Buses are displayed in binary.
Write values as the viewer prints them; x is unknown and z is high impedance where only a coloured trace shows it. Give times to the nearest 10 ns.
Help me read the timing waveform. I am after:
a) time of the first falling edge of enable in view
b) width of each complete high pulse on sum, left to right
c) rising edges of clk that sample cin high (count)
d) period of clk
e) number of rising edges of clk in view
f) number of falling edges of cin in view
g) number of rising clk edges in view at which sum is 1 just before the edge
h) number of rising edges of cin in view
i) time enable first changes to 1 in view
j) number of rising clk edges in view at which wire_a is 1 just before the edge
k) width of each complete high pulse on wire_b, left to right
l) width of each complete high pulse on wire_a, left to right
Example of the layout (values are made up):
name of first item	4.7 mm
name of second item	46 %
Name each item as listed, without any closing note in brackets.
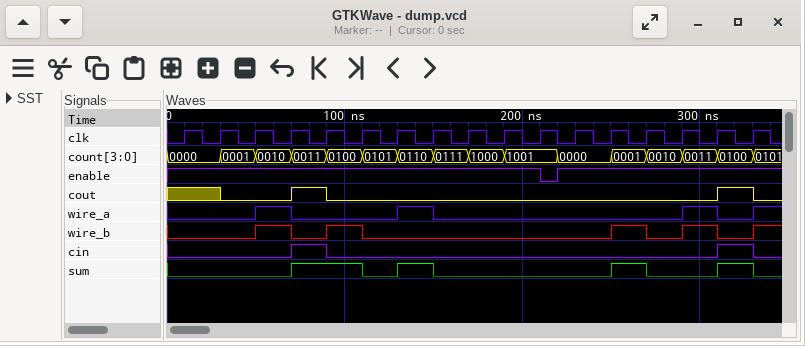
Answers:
time of the first falling edge of enable in view	210 ns
width of each complete high pulse on sum, left to right	40 ns, 20 ns, 20 ns, 20 ns
rising edges of clk that sample cin high	2
period of clk	20 ns
number of rising edges of clk in view	17
number of falling edges of cin in view	2
number of rising clk edges in view at which sum is 1 just before the edge	5
number of rising edges of cin in view	2
time enable first changes to 1 in view	220 ns
number of rising clk edges in view at which wire_a is 1 just before the edge	3
width of each complete high pulse on wire_b, left to right	20 ns, 20 ns, 20 ns, 20 ns
width of each complete high pulse on wire_a, left to right	20 ns, 20 ns, 20 ns
